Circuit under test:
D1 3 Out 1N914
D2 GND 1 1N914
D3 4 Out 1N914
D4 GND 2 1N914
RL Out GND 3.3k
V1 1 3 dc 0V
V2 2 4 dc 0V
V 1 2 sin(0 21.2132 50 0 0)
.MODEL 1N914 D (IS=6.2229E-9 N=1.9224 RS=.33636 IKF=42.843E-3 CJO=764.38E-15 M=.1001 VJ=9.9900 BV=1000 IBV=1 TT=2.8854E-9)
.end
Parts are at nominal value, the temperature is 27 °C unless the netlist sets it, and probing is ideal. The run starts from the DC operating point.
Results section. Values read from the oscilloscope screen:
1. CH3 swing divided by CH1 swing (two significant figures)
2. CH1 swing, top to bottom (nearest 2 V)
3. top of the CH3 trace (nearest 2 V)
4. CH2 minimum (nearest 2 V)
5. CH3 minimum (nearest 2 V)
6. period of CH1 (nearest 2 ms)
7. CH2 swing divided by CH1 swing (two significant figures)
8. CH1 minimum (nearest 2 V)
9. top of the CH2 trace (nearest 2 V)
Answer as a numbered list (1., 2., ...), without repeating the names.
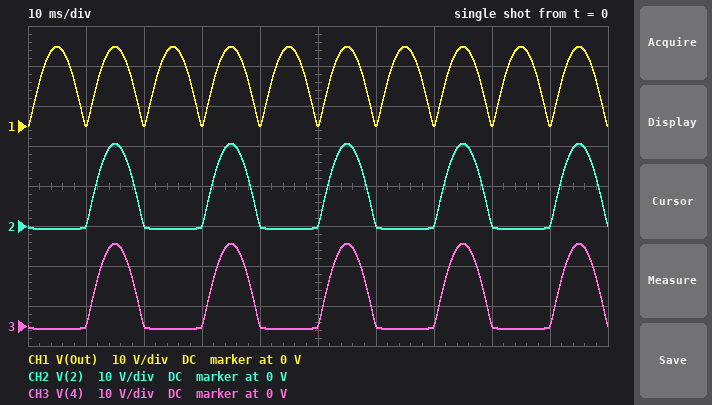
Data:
1. 1.1
2. 20 V
3. 20 V
4. 0 V
5. 0 V
6. 10 ms
7. 1.1
8. 0 V
9. 20 V
